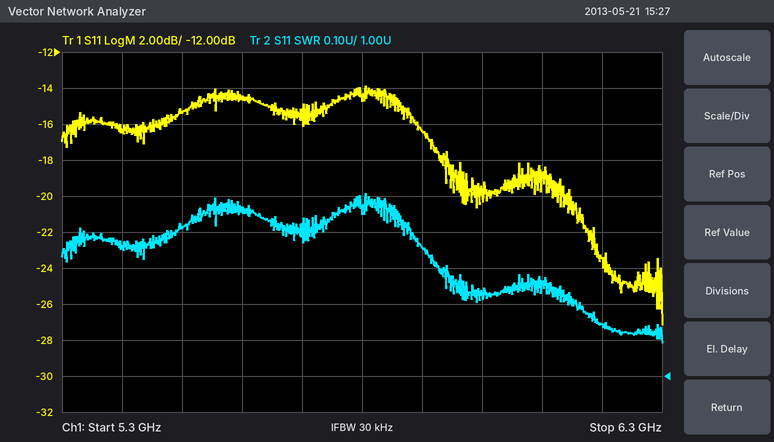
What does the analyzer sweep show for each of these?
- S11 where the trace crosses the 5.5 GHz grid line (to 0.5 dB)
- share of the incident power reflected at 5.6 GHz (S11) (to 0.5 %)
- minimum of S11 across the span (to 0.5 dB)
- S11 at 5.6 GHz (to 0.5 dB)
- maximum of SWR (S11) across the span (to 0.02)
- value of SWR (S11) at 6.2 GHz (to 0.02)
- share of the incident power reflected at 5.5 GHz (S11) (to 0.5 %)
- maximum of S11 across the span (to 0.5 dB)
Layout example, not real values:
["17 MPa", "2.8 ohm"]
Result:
["-15.5 dB", "3.5 %", "-27.0 dB", "-14.5 dB", "1.50", "1.14", "3.0 %", "-14.0 dB"]
